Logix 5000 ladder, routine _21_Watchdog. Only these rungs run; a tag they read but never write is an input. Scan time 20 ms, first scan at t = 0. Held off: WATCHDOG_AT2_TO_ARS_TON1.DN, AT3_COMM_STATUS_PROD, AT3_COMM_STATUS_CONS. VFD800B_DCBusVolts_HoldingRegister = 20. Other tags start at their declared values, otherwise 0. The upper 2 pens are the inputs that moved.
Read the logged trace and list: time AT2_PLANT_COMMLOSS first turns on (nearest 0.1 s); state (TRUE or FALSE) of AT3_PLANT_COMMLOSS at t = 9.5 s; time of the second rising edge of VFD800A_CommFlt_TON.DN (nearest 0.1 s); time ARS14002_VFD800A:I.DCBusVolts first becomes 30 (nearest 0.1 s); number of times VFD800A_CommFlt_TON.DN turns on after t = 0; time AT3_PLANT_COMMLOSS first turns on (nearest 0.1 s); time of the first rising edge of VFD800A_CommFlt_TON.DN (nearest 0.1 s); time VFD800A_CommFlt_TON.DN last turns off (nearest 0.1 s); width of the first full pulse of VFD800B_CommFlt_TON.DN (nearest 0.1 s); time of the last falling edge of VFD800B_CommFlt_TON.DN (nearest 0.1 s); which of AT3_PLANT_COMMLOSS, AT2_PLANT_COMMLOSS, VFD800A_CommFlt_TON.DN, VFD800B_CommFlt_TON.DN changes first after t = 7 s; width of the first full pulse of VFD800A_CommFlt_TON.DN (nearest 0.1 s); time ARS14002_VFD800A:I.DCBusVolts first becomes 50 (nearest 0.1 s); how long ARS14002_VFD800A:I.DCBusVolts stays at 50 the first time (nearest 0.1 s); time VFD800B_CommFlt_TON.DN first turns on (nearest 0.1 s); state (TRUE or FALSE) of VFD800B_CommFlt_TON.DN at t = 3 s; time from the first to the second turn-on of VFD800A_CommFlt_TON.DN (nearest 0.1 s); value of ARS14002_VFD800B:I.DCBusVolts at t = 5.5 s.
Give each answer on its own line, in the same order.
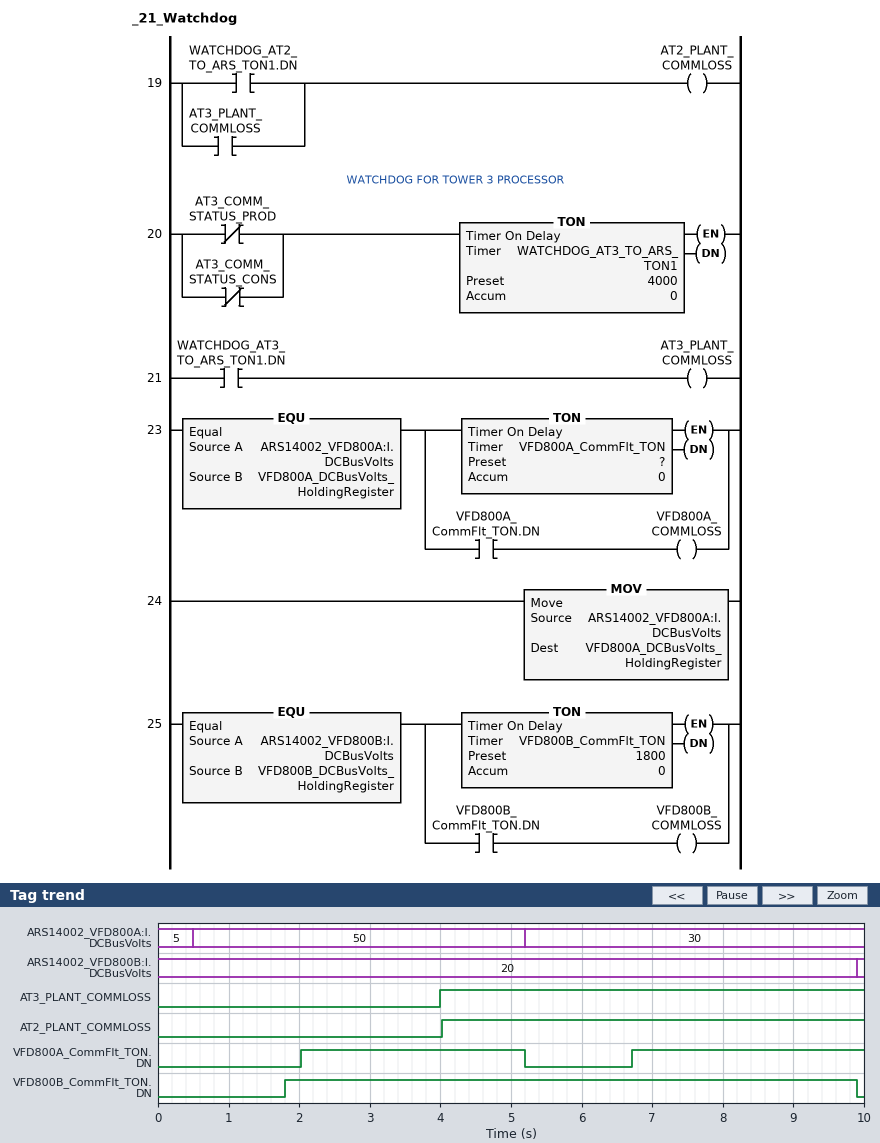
4.0 s
TRUE
6.7 s
5.2 s
2
4.0 s
2.0 s
5.2 s
8.1 s
9.9 s
VFD800B_CommFlt_TON.DN
3.2 s
0.5 s
4.7 s
1.8 s
TRUE
4.7 s
20
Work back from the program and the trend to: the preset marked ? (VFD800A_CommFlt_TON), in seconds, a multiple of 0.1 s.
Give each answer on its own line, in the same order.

1.5 s
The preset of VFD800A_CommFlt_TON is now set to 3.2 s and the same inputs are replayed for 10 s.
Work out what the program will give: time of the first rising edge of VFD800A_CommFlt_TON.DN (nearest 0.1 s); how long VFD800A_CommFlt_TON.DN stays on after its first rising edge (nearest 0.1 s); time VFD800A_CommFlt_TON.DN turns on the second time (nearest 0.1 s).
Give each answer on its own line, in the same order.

3.7 s
1.5 s
8.4 s
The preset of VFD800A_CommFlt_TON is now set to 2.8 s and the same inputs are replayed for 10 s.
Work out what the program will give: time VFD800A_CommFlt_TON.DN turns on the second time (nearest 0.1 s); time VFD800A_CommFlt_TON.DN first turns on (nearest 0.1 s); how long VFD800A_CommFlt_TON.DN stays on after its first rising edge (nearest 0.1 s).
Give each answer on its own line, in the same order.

8.0 s
3.3 s
1.9 s
